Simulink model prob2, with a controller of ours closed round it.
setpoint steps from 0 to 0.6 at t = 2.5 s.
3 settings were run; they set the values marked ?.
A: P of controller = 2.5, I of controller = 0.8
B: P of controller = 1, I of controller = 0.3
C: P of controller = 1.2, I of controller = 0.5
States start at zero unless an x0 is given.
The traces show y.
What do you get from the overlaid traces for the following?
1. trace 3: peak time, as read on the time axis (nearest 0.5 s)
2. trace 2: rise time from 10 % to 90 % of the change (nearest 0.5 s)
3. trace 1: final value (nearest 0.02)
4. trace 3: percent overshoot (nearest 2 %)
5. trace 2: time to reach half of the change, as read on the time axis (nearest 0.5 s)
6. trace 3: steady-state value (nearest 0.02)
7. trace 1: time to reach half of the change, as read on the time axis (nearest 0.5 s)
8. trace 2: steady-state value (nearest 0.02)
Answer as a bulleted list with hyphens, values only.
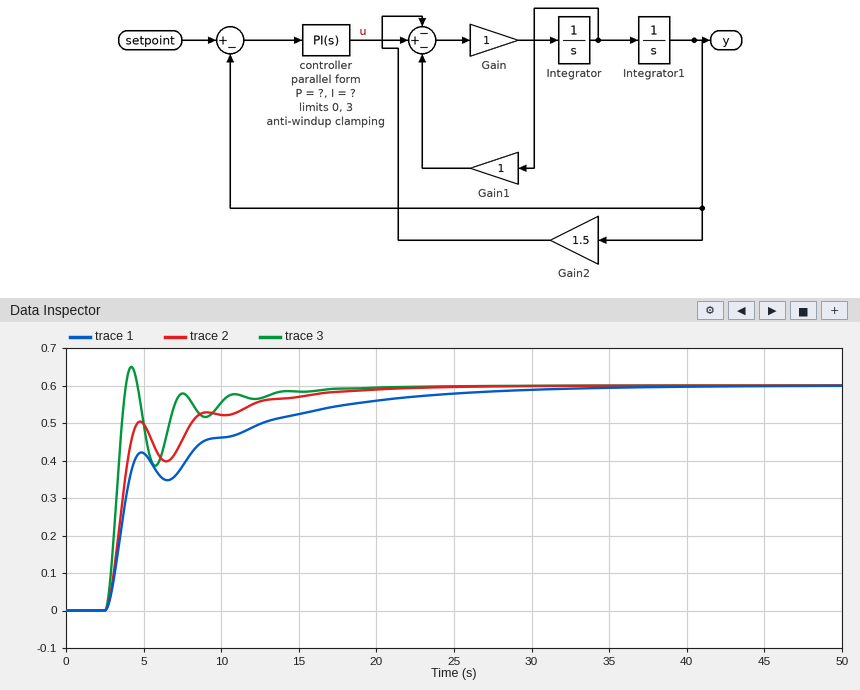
- 4.0 s
- 8.5 s
- 0.60
- 8 %
- 3.5 s
- 0.60
- 4.0 s
- 0.60
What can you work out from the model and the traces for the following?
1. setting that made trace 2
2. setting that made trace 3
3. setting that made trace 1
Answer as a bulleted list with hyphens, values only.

- C
- A
- B
